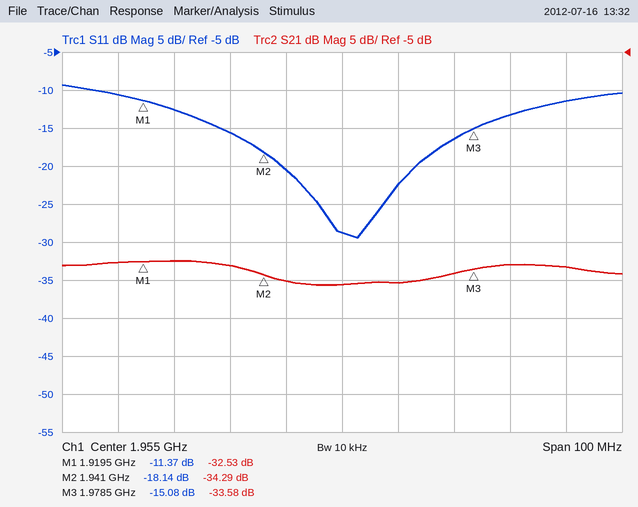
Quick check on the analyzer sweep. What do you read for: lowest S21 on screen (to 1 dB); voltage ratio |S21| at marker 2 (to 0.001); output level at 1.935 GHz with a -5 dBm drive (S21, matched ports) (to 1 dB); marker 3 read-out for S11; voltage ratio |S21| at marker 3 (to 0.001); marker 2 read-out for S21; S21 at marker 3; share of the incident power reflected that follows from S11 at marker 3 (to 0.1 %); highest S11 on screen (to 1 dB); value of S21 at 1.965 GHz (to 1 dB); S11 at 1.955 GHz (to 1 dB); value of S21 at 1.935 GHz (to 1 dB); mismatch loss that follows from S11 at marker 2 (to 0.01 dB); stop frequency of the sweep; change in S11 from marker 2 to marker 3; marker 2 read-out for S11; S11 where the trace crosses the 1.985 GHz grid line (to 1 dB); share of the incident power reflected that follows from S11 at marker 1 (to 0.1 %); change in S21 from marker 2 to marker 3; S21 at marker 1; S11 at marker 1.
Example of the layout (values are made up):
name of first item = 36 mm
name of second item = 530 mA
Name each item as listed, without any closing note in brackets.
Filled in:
lowest S21 on screen = -36 dB
voltage ratio |S21| at marker 2 = 0.019
output level at 1.935 GHz with a -5 dBm drive (S21, matched ports) = -38 dBm
marker 3 read-out for S11 = -15.08 dB
voltage ratio |S21| at marker 3 = 0.021
marker 2 read-out for S21 = -34.29 dB
S21 at marker 3 = -33.58 dB
share of the incident power reflected that follows from S11 at marker 3 = 3.1 %
highest S11 on screen = -9 dB
value of S21 at 1.965 GHz = -35 dB
S11 at 1.955 GHz = -29 dB
value of S21 at 1.935 GHz = -33 dB
mismatch loss that follows from S11 at marker 2 = 0.07 dB
stop frequency of the sweep = 2.005 GHz
change in S11 from marker 2 to marker 3 = 3.06 dB
marker 2 read-out for S11 = -18.14 dB
S11 where the trace crosses the 1.985 GHz grid line = -13 dB
share of the incident power reflected that follows from S11 at marker 1 = 7.3 %
change in S21 from marker 2 to marker 3 = 0.71 dB
S21 at marker 1 = -32.53 dB
S11 at marker 1 = -11.37 dB
